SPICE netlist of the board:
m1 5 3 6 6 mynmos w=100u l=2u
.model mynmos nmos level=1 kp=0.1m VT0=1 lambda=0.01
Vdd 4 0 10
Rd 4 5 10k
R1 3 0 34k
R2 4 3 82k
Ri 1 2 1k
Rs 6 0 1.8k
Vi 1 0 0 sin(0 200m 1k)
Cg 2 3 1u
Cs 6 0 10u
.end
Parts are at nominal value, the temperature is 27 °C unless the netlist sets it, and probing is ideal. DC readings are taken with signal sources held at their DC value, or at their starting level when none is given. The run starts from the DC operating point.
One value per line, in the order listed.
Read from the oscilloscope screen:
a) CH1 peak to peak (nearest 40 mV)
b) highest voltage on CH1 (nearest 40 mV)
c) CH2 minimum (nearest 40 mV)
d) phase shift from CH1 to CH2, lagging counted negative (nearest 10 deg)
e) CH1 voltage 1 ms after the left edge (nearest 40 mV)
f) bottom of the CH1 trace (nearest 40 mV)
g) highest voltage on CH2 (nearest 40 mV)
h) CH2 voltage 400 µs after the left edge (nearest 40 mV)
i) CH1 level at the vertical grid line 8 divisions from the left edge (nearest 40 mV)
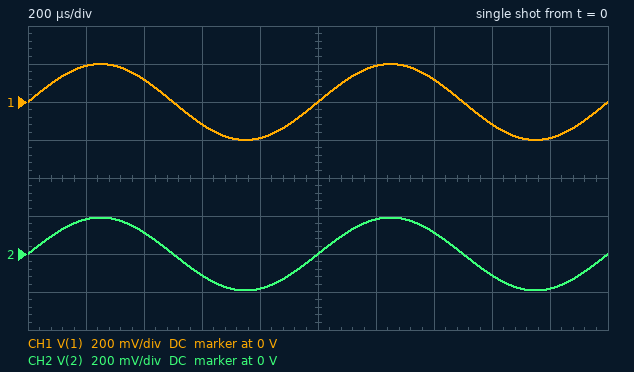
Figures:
400 mV
200 mV
-200 mV
0 deg
0 V
-200 mV
200 mV
120 mV
-120 mV
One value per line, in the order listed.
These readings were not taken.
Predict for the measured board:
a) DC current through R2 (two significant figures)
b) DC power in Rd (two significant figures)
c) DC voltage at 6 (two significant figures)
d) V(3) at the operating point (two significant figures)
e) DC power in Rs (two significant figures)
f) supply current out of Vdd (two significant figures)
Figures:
86 µA
5.9 mW
1.4 V
2.9 V
1.1 mW
850 µA
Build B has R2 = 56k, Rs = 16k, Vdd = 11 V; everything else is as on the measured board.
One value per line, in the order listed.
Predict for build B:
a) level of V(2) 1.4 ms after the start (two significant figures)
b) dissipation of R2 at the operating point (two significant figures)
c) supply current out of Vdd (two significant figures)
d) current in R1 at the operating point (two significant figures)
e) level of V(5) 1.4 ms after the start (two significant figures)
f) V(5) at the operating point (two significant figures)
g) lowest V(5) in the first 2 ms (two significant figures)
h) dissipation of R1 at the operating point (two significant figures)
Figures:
110 mV
840 µW
300 µA
120 µA
7.6 V
9.2 V
5.9 V
510 µW
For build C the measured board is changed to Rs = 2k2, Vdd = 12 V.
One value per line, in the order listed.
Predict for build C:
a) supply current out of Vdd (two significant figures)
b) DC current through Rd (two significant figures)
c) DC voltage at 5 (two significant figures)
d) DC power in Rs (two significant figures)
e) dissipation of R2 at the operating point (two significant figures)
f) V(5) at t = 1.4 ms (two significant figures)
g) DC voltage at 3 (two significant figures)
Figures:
980 µA
880 µA
3.2 V
1.7 mW
880 µW
2.3 V
3.5 V
